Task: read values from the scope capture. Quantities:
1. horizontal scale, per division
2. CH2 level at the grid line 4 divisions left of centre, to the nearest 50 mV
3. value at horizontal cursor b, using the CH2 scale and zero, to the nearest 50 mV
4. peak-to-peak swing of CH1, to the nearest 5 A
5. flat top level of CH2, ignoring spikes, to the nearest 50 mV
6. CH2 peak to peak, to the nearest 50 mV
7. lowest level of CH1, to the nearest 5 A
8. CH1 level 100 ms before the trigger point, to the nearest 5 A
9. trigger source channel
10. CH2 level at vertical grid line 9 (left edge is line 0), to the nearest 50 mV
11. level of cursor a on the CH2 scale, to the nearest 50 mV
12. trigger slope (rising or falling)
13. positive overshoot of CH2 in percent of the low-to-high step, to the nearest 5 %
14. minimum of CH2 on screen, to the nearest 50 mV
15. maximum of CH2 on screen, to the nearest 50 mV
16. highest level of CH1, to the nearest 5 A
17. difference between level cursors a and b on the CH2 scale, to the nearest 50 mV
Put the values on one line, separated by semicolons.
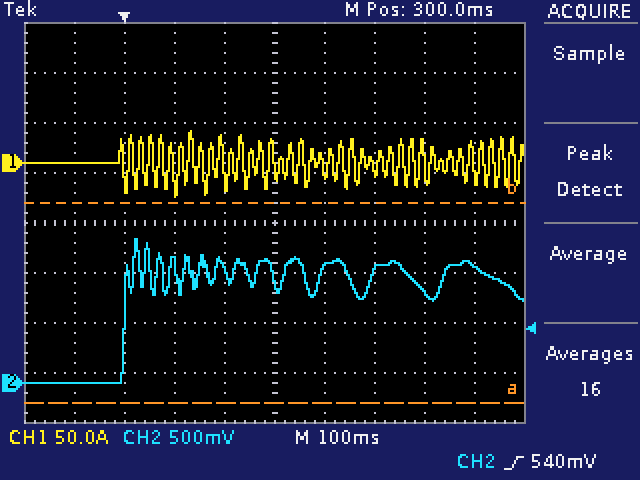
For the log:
100 ms; 0 mV; 1.80 V; 65 A; 1.20 V; 1.45 V; -35 A; 0 A; CH2; 1.15 V; -200 mV; rising; 20 %; 0 mV; 1.45 V; 30 A; 2.00 V
